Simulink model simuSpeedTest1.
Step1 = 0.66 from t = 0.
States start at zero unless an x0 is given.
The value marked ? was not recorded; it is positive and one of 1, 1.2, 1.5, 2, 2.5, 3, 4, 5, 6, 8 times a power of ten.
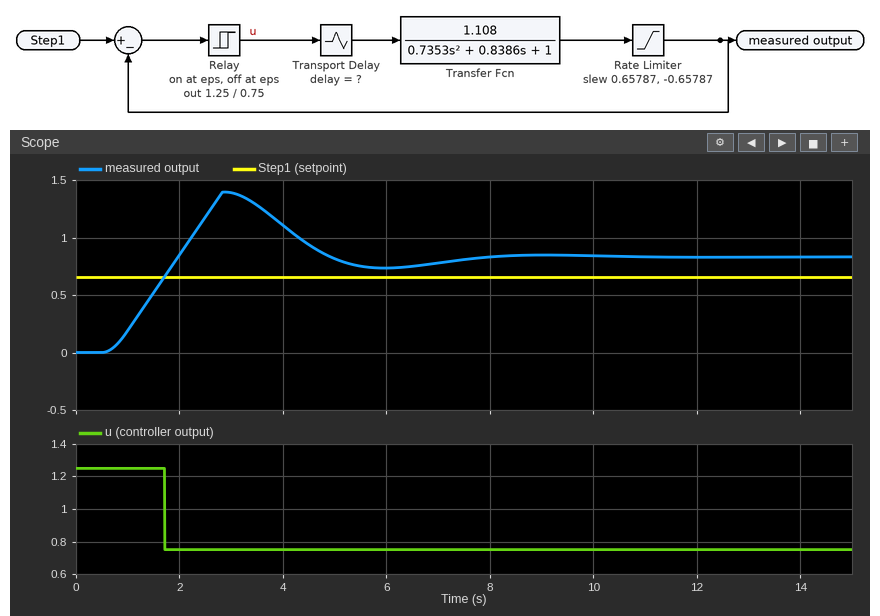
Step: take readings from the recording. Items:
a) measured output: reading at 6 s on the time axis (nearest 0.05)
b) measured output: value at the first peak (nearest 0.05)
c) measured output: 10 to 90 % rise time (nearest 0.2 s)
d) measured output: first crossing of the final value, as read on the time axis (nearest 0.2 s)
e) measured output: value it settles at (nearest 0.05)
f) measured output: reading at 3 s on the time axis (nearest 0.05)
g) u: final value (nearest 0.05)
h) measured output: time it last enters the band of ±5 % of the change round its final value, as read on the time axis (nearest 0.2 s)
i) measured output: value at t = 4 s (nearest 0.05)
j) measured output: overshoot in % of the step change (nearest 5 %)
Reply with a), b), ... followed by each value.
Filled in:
a) 0.75
b) 1.40
c) 1.0 s
d) 2.0 s
e) 0.85
f) 1.40
g) 0.75
h) 7.2 s
i) 1.10
j) 70 %
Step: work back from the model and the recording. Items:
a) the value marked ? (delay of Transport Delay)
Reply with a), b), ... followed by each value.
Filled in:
a) 0.5
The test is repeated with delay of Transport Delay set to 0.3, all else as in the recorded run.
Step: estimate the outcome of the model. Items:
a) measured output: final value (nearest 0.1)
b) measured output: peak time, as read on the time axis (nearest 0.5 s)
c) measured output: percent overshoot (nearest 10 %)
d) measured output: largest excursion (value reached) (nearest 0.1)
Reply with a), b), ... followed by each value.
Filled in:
a) 0.8
b) 2.5 s
c) 60 %
d) 1.3
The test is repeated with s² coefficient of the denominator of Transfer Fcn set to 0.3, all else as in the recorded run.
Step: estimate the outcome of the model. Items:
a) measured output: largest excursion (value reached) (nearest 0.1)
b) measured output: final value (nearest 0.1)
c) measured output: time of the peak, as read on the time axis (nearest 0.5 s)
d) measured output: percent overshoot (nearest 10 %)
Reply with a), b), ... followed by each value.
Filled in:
a) 1.3
b) 0.8
c) 2.5 s
d) 50 %
